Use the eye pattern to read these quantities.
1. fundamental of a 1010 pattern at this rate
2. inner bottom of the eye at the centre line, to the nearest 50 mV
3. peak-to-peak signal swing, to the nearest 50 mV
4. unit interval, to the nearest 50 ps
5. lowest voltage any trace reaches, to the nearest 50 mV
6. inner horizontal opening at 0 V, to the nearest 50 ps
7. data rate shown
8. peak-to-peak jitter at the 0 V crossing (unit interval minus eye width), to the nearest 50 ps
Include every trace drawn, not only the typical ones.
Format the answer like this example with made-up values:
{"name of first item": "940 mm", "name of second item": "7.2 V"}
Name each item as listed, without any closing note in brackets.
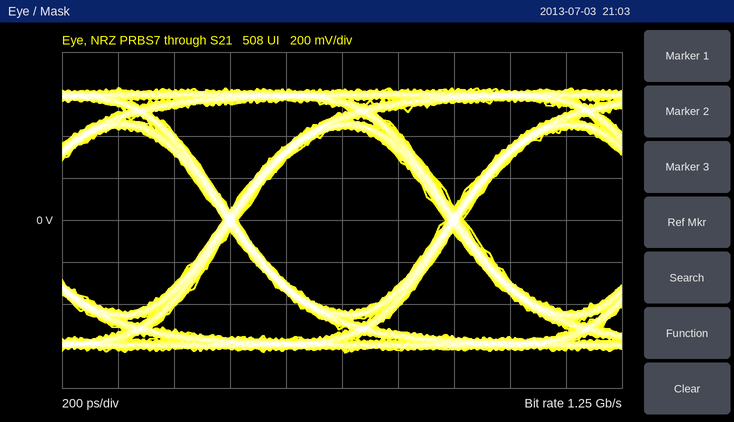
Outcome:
{"fundamental of a 1010 pattern at this rate": "625 MHz", "inner bottom of the eye at the centre line, to the nearest 50 mV": "-450 mV", "peak-to-peak signal swing, to the nearest 50 mV": "1.25 V", "unit interval, to the nearest 50 ps": "800 ps", "lowest voltage any trace reaches, to the nearest 50 mV": "-650 mV", "inner horizontal opening at 0 V, to the nearest 50 ps": "750 ps", "data rate shown": "1.25 Gb/s", "peak-to-peak jitter at the 0 V crossing (unit interval minus eye width), to the nearest 50 ps": "50 ps"}
